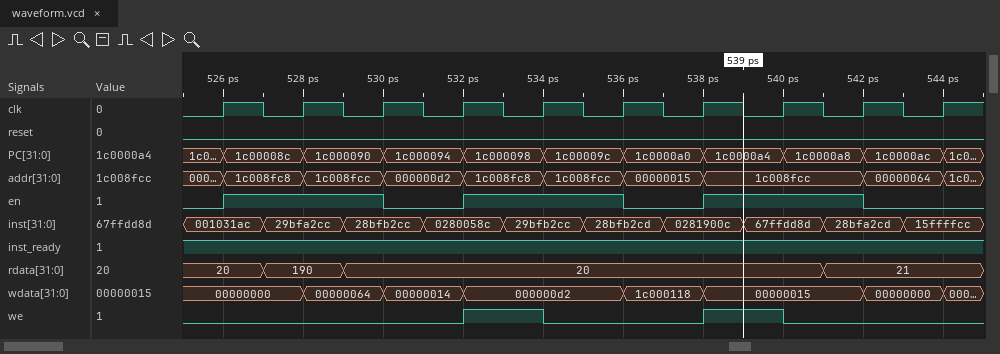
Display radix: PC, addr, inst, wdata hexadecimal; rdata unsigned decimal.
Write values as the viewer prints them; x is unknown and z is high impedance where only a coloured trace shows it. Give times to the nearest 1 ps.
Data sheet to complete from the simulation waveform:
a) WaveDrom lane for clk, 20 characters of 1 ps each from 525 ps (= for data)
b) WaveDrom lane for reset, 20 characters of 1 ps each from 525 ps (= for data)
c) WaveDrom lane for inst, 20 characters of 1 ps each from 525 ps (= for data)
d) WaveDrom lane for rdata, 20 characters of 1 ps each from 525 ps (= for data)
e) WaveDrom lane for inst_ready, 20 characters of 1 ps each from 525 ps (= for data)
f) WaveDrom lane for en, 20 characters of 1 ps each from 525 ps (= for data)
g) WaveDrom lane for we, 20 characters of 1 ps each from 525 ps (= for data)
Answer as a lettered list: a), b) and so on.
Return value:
a) {name: 'clk', wave: '01010101010101010101'}
b) {name: 'reset', wave: '0...................'}
c) {name: 'inst', wave: '=.=.=.=.=.=.=.=.=.=.', data: '001031ac 29bfa2cc 28bfb2cc 0280058c 29bfb2cc 28bfb2cd 0281900c 67ffdd8d 28bfa2cd 15ffffcc'}
d) {name: 'rdata', wave: '=.=.=...........=...', data: '20 190 20 21'}
e) {name: 'inst_ready', wave: '1...................'}
f) {name: 'en', wave: '01...0.1...0.1...0..'}
g) {name: 'we', wave: '0......1.0...1.0....'}
